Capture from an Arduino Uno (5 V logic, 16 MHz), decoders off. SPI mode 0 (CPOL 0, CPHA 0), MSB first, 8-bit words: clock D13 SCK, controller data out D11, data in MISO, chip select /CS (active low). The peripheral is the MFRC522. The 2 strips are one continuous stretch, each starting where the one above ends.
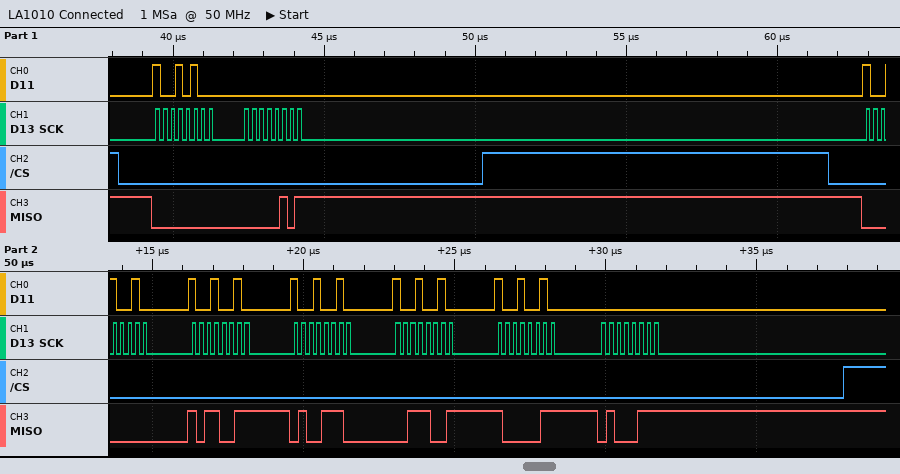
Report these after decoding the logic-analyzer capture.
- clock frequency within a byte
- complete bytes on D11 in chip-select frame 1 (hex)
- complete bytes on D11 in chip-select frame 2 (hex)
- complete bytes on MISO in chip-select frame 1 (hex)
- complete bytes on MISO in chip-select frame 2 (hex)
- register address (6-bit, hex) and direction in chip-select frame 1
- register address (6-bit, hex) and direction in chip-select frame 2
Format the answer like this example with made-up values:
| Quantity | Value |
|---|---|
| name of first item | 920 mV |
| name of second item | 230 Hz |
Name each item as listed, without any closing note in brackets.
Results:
| Quantity | Value |
|---|---|
| clock frequency within a byte | 4 MHz |
| complete bytes on D11 in chip-select frame 1 | 94 00 |
| complete bytes on D11 in chip-select frame 2 | 92 92 92 92 92 00 |
| complete bytes on MISO in chip-select frame 1 | 00 05 |
| complete bytes on MISO in chip-select frame 2 | 00 B3 4E 39 83 47 |
| register address (6-bit, hex) and direction in chip-select frame 1 | 0x0A read |
| register address (6-bit, hex) and direction in chip-select frame 2 | 0x09 read |
